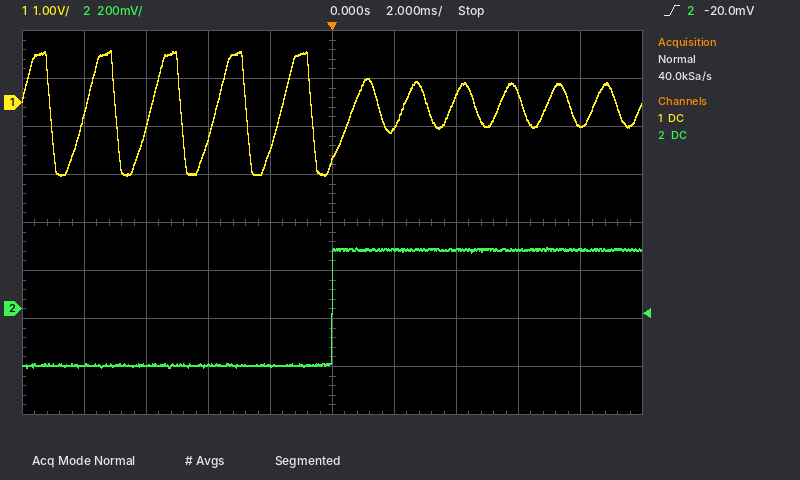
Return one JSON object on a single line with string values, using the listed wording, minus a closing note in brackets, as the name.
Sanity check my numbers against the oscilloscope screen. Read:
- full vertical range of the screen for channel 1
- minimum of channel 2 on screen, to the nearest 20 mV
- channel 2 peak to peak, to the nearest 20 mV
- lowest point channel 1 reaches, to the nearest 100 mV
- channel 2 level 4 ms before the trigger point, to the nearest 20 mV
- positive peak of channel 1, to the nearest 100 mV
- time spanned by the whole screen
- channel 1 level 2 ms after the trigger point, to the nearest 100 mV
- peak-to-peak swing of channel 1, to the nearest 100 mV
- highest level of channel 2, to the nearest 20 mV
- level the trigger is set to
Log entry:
{"full vertical range of the screen for channel 1": "8 V", "minimum of channel 2 on screen, to the nearest 20 mV": "-240 mV", "channel 2 peak to peak, to the nearest 20 mV": "500 mV", "lowest point channel 1 reaches, to the nearest 100 mV": "-1.5 V", "channel 2 level 4 ms before the trigger point, to the nearest 20 mV": "-240 mV", "positive peak of channel 1, to the nearest 100 mV": "1.1 V", "time spanned by the whole screen": "20 ms", "channel 1 level 2 ms after the trigger point, to the nearest 100 mV": "-500 mV", "peak-to-peak swing of channel 1, to the nearest 100 mV": "2.6 V", "highest level of channel 2, to the nearest 20 mV": "260 mV", "level the trigger is set to": "-20.0 mV"}
